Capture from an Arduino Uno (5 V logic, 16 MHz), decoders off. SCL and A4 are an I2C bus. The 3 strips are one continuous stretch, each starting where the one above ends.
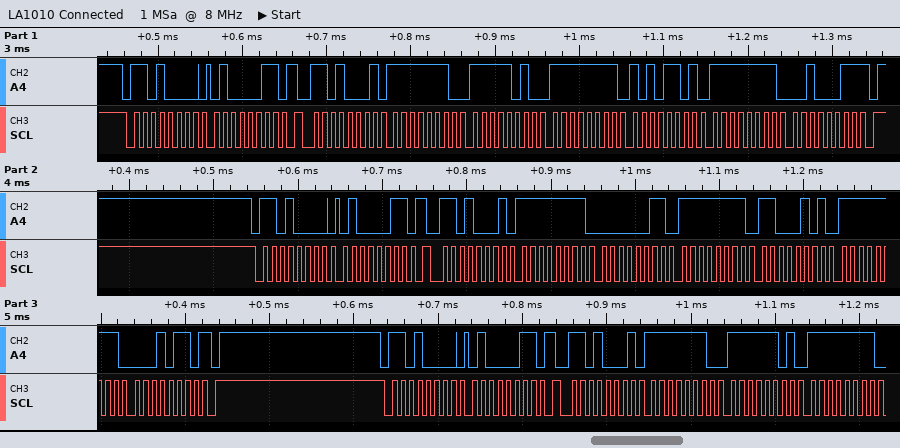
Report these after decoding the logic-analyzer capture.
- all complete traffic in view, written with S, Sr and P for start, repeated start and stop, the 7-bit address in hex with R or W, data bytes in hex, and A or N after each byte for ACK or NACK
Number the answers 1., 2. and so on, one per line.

1. S 68W A 43 A Sr 68R A FE A FA A FF A AD A FF A 23 N P S 68W A 43 A Sr 68R A FF A 03 A FF A C5 A FF A 16 N P S 68W A 43 A Sr 68R A FE A FD A FF A
